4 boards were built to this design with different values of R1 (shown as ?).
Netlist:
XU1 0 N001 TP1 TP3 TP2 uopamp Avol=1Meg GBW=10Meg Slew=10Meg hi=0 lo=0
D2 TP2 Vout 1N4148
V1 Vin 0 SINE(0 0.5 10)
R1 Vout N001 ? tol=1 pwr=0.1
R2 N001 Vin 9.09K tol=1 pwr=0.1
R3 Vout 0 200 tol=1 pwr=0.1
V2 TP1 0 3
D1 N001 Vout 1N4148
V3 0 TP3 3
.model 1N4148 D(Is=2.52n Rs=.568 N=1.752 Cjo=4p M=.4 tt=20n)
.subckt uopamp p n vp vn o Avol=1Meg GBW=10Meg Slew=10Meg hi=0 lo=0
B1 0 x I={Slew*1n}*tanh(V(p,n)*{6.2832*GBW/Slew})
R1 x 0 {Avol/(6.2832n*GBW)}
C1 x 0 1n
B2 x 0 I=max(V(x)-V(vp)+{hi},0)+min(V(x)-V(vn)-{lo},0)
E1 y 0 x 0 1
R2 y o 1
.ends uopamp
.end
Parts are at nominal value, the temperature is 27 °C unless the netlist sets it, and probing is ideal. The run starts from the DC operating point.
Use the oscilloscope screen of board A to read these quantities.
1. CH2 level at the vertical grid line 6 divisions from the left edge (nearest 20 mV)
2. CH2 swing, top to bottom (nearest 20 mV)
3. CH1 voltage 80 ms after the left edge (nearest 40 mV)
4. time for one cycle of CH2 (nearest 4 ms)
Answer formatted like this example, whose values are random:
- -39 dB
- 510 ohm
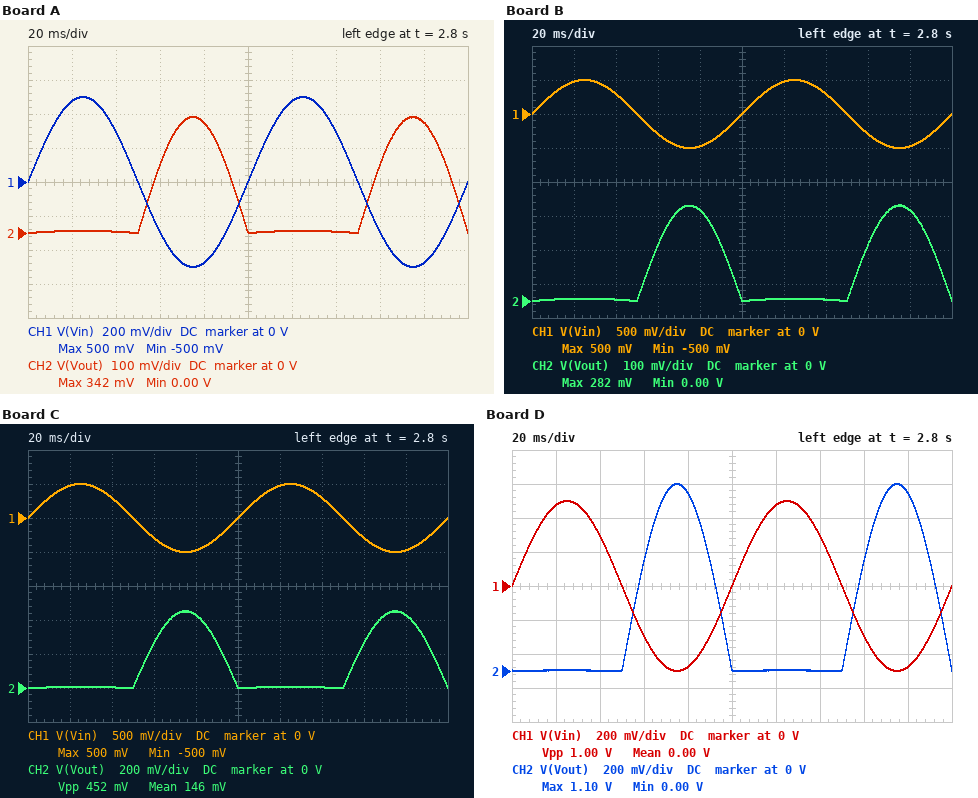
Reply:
- 0 V
- 340 mV
- -480 mV
- 100 ms
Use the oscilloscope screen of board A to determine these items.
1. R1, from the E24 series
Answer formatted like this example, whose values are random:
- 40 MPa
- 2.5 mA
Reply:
- 6.2 kΩ
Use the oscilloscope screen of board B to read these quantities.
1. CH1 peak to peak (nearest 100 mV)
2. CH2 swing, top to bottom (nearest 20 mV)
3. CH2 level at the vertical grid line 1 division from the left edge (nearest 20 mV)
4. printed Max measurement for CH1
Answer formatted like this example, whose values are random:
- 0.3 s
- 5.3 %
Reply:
- 1.0 V
- 280 mV
- 0 V
- 500 mV
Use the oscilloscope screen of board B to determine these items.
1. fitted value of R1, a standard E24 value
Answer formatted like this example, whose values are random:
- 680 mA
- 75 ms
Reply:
- 5.1 kΩ
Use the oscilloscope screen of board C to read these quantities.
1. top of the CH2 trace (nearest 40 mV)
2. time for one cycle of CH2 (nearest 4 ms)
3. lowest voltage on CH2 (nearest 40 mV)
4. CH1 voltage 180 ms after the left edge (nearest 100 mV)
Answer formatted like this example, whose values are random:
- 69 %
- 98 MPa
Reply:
- 440 mV
- 100 ms
- 0 V
- -500 mV
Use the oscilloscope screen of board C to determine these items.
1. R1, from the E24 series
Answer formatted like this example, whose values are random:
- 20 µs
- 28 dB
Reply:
- 8.2 kΩ
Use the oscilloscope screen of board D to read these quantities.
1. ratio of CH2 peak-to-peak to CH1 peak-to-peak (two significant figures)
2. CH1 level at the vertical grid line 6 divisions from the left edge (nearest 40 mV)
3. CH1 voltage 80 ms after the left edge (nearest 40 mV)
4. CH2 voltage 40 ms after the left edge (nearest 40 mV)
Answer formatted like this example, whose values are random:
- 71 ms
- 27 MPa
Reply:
- 1.1
- 480 mV
- -480 mV
- 0 V
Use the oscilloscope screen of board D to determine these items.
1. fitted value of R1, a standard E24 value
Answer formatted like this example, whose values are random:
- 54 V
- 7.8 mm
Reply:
- 20 kΩ
